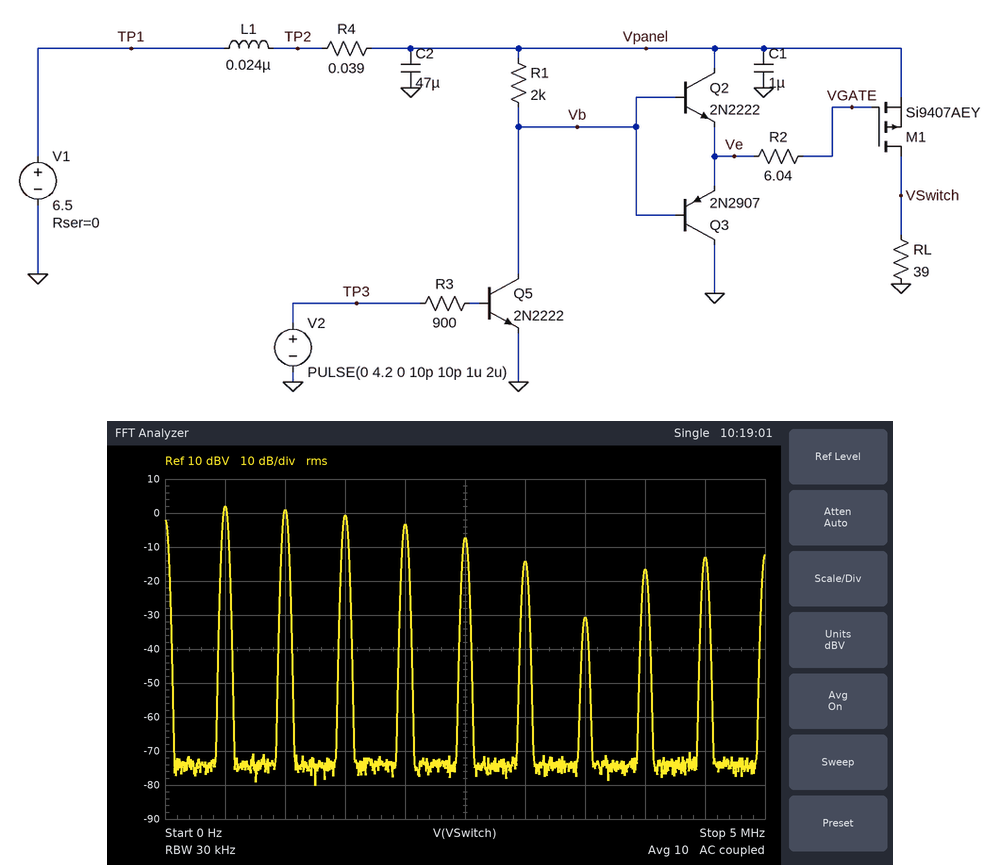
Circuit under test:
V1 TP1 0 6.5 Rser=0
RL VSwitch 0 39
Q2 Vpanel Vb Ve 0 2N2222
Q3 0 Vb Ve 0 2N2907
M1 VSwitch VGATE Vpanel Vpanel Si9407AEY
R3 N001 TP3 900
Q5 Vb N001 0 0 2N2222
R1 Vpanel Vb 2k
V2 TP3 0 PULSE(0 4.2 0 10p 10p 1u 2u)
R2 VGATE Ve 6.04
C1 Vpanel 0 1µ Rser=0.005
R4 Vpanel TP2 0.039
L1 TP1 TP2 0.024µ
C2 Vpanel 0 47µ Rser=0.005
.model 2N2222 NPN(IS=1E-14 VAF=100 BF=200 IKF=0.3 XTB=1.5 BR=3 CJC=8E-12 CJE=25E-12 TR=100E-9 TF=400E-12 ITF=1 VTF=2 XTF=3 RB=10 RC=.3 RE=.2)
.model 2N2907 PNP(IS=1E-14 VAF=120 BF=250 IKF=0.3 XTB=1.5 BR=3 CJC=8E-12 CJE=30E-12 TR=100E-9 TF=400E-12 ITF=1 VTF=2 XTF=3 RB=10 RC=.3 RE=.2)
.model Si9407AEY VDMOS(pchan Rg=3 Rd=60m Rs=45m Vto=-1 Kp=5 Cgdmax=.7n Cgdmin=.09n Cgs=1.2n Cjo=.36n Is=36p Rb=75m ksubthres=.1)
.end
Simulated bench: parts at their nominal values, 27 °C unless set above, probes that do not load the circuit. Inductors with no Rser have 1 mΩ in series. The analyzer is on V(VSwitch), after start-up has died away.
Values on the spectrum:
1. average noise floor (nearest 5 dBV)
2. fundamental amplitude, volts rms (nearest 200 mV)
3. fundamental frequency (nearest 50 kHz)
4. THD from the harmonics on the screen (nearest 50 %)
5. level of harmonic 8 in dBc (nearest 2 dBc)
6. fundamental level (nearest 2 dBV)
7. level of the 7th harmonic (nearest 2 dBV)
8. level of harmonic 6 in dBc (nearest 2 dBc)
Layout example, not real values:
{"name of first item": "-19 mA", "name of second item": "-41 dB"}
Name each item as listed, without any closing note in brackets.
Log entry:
{"average noise floor": "-75 dBV", "fundamental amplitude, volts rms": "1.2 V", "fundamental frequency": "500 kHz", "THD from the harmonics on the screen": "150 %", "level of harmonic 8 in dBc": "-18 dBc", "fundamental level": "2 dBV", "level of the 7th harmonic": "-30 dBV", "level of harmonic 6 in dBc": "-16 dBc"}
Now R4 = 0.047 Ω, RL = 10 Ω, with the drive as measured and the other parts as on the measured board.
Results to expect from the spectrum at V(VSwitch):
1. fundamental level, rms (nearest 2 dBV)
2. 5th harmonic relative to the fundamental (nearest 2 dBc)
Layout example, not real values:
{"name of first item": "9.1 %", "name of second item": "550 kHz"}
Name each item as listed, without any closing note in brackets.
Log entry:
{"fundamental level, rms": "2 dBV", "5th harmonic relative to the fundamental": "-12 dBc"}
